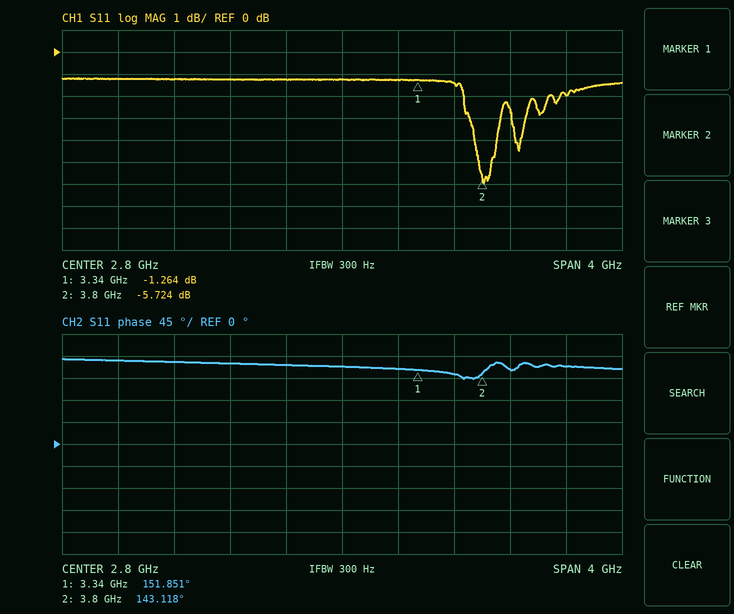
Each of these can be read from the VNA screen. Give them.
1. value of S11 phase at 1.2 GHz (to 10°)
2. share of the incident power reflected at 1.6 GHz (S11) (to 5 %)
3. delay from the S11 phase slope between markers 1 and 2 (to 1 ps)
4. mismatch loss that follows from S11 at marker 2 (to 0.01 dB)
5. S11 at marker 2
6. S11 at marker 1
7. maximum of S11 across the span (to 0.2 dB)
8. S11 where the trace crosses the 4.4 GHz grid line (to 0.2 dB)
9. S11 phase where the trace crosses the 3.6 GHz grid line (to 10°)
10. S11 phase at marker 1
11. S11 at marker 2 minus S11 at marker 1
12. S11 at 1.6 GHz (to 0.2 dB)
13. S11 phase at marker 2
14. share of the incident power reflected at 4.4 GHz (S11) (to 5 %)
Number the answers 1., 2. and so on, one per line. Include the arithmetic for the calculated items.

1. 170°
2. 10^(-1.2/10) ≈ 75.9 %, so 75 % to the nearest 5 %
3. −(143.118° − (151.851°))/(360° × 460 MHz) ≈ 53 ps
4. −10 log10(1 − 10^(-5.724/10)) ≈ 1.35 dB
5. -5.724 dB
6. -1.264 dB
7. -1.2 dB
8. -2.0 dB
9. 140°
10. 151.851°
11. -5.724 − (-1.264) = -4.460 dB
12. -1.2 dB
13. 143.118°
14. 10^(-2/10) ≈ 63.1 %, so 65 % to the nearest 5 %
